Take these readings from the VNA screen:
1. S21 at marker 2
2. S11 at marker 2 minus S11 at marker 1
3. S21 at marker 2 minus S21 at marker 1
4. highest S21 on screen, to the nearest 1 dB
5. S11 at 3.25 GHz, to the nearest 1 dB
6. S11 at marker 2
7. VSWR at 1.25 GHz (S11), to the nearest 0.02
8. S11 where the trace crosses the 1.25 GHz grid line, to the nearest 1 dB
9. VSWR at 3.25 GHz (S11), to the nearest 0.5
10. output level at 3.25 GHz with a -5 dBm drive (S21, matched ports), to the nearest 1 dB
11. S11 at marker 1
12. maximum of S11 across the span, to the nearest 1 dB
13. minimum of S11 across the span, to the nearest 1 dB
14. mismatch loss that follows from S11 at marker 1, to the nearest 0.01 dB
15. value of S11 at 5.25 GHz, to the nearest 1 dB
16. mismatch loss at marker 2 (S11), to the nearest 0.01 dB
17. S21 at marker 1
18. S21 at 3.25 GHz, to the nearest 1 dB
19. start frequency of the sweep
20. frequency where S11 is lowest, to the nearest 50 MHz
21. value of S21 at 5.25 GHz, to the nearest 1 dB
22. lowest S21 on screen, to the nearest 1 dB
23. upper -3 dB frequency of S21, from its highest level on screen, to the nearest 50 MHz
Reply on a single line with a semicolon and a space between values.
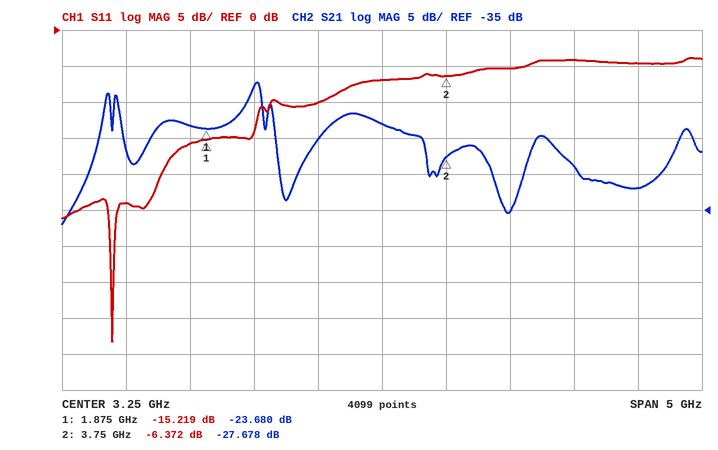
-27.678 dB; 8.847 dB; -3.998 dB; -17 dB; -7 dB; -6.372 dB; 1.14; -24 dB; 2.5; -28 dBm; -15.219 dB; -4 dB; -43 dB; 0.13 dB; -5 dB; 1.14 dB; -23.680 dB; -23 dB; 750 MHz; 1.15 GHz; -32 dB; -37 dB; 2.30 GHz
